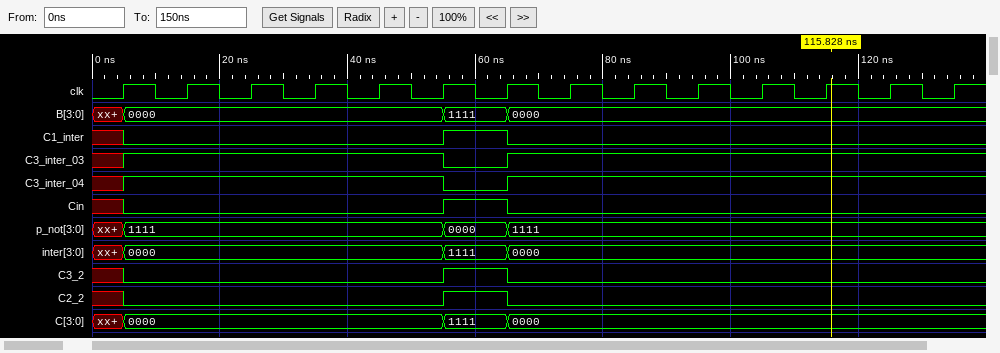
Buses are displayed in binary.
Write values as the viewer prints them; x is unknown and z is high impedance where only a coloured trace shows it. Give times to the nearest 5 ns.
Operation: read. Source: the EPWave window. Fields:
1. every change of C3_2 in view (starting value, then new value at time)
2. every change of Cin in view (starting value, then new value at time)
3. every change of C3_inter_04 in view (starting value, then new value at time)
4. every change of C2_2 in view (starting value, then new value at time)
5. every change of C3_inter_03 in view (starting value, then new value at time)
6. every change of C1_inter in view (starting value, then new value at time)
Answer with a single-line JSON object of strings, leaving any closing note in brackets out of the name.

{"every change of C3_2 in view": "x, 0 at 5 ns, 1 at 55 ns, 0 at 65 ns", "every change of Cin in view": "x, 0 at 5 ns, 1 at 55 ns, 0 at 65 ns", "every change of C3_inter_04 in view": "x, 1 at 5 ns, 0 at 55 ns, 1 at 65 ns", "every change of C2_2 in view": "x, 0 at 5 ns, 1 at 55 ns, 0 at 65 ns", "every change of C3_inter_03 in view": "x, 1 at 5 ns, 0 at 55 ns, 1 at 65 ns", "every change of C1_inter in view": "x, 0 at 5 ns, 1 at 55 ns, 0 at 65 ns"}
